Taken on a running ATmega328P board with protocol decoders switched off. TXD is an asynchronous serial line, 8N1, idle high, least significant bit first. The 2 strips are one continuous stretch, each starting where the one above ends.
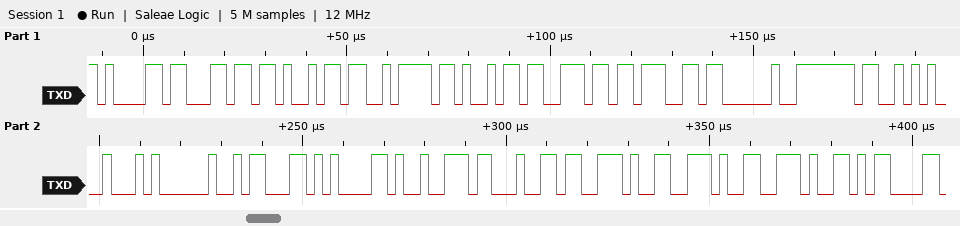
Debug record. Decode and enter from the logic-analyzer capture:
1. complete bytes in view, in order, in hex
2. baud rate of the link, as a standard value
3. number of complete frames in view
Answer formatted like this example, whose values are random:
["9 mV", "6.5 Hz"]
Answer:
["61 6C 69 7A 69 6E 67 20 53 44 20 63 61 72 64 2E 2E 2E 0D", "500000 baud", "19"]
